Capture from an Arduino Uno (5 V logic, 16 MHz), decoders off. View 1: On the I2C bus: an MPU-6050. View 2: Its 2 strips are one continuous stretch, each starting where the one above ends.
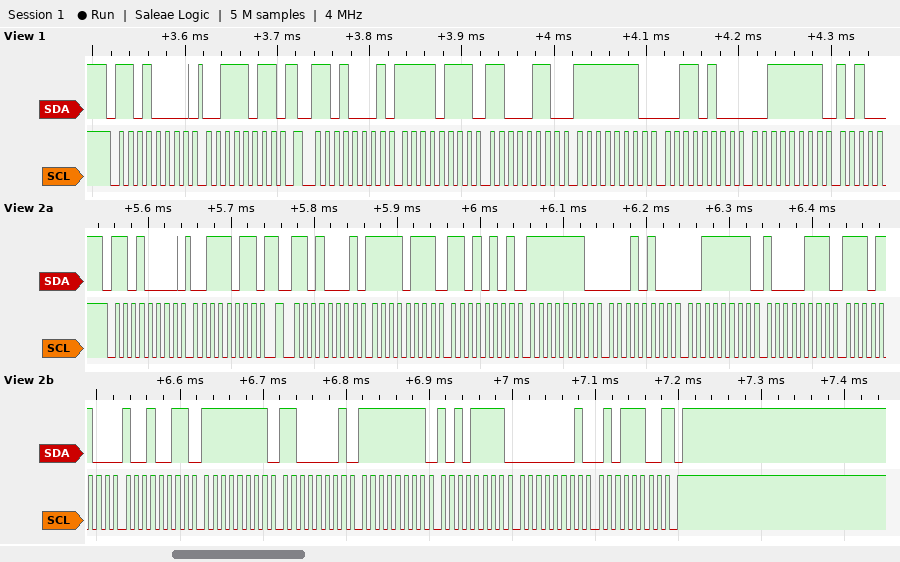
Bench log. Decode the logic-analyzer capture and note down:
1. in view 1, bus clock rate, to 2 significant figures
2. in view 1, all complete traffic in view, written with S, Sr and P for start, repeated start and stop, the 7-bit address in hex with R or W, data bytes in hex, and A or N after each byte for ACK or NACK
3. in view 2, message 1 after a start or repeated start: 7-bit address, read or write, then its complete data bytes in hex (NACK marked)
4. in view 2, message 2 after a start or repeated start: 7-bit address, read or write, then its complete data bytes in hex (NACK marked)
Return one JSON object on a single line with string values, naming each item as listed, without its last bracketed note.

{"in view 1, bus clock rate, to 2 significant figures": "100 kHz", "in view 1, all complete traffic in view, written with S, Sr and P for start, repeated start and stop, the 7-bit address in hex with R or W, data bytes in hex, and A or N after each byte for ACK or NACK": "S 68W A 3B A Sr 68R A F7 A C6 A FE A 34 A 3F A", "in view 2, message 1 after a start or repeated start: 7-bit address, read or write, then its complete data bytes in hex": "0x68 write: 3B", "in view 2, message 2 after a start or repeated start: 7-bit address, read or write, then its complete data bytes in hex": "0x68 read: F7 D5 FE 14 3F 87 EC 93 FF C1 FF AF 01 5C NACK"}
